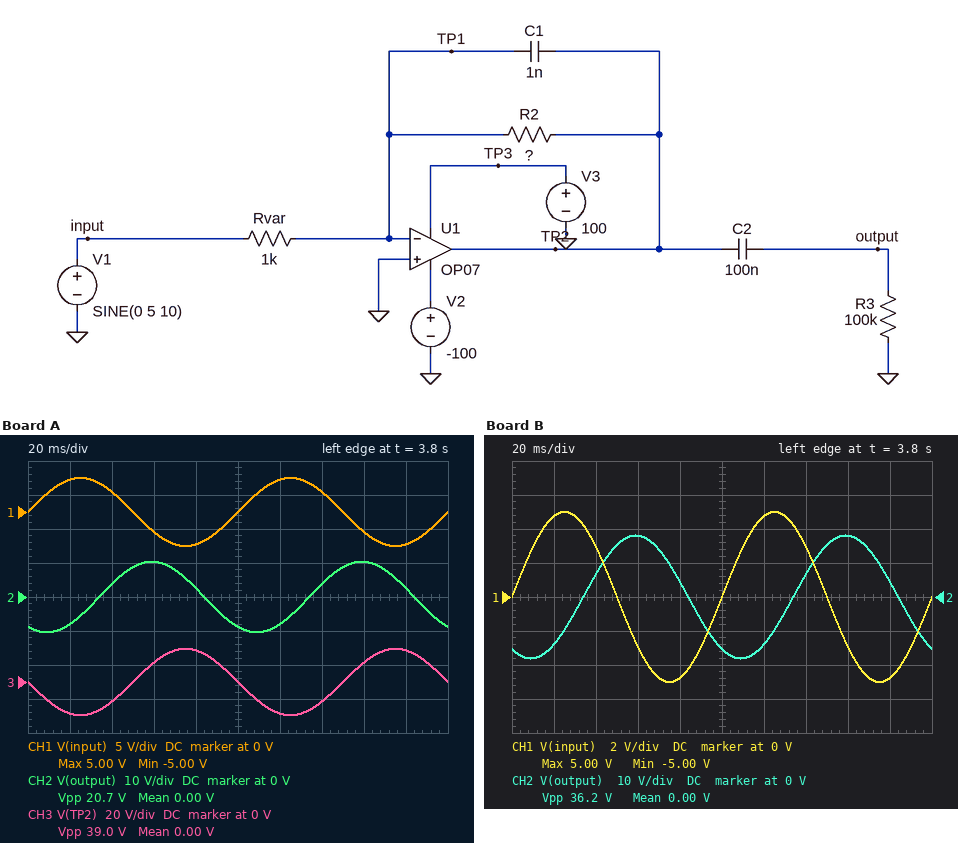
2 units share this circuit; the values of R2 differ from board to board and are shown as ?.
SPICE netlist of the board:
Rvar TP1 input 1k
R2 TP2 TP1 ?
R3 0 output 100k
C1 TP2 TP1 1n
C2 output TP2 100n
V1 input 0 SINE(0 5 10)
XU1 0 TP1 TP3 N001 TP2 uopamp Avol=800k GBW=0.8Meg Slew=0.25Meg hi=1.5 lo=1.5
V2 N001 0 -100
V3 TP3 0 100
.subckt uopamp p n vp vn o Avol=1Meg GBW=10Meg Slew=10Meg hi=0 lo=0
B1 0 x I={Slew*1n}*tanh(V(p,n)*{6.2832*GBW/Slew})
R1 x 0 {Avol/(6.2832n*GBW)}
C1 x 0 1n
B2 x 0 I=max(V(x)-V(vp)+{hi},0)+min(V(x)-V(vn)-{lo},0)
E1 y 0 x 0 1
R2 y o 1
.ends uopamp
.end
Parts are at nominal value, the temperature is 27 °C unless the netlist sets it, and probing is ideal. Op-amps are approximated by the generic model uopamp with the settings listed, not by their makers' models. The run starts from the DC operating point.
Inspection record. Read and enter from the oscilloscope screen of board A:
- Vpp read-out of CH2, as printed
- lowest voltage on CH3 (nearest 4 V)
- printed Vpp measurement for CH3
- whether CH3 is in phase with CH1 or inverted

20.7 V
-20 V
39.0 V
inverted
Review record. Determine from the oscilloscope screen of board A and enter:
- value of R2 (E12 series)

3.9 kΩ
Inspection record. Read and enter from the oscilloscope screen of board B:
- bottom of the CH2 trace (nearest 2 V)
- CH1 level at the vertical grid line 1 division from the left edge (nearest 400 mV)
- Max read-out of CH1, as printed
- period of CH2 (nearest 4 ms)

-18 V
4.8 V
5.00 V
100 ms
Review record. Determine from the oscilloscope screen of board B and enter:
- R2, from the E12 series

6.8 kΩ
